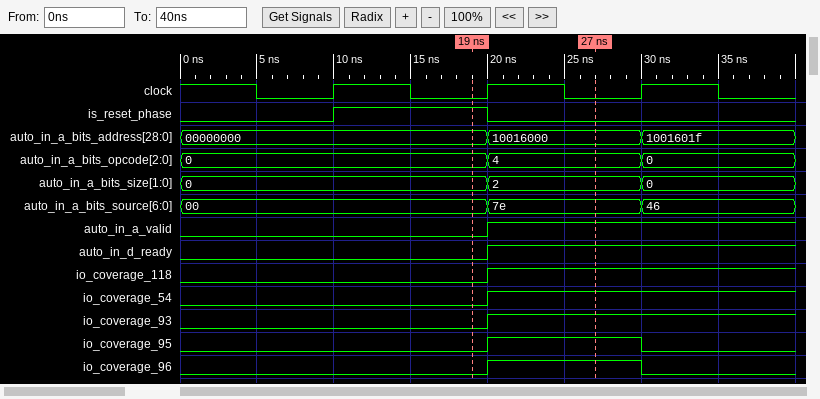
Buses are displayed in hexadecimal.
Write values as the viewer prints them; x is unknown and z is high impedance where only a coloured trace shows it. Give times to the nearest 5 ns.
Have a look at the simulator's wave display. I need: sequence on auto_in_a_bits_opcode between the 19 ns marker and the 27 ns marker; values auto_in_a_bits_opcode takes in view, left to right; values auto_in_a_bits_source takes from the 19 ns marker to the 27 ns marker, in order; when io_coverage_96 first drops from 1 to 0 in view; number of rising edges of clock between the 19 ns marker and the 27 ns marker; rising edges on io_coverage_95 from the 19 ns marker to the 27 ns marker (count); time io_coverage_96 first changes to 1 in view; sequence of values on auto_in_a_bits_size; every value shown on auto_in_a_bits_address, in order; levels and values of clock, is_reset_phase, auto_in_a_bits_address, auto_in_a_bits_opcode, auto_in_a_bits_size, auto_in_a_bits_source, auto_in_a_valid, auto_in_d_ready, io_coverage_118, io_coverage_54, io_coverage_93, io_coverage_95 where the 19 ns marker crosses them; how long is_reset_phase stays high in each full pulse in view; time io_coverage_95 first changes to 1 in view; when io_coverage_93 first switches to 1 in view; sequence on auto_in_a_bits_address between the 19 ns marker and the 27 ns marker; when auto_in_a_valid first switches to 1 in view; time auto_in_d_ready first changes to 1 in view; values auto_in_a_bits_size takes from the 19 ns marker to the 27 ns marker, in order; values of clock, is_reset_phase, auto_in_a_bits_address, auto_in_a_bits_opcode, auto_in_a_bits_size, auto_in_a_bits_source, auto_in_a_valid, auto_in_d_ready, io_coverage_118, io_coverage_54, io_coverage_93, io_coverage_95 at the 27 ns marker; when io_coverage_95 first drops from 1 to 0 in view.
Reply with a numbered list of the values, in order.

1. 0, 4
2. 0, 4, 0
3. 00, 7e
4. 30 ns
5. 1
6. 1
7. 20 ns
8. 0, 2, 0
9. 00000000, 10016000, 1001601f
10. clock=0, is_reset_phase=1, auto_in_a_bits_address=00000000, auto_in_a_bits_opcode=0, auto_in_a_bits_size=0, auto_in_a_bits_source=00, auto_in_a_valid=0, auto_in_d_ready=0, io_coverage_118=0, io_coverage_54=0, io_coverage_93=0, io_coverage_95=0
11. 10 ns
12. 20 ns
13. 20 ns
14. 00000000, 10016000
15. 20 ns
16. 20 ns
17. 0, 2
18. clock=0, is_reset_phase=0, auto_in_a_bits_address=10016000, auto_in_a_bits_opcode=4, auto_in_a_bits_size=2, auto_in_a_bits_source=7e, auto_in_a_valid=1, auto_in_d_ready=1, io_coverage_118=1, io_coverage_54=1, io_coverage_93=1, io_coverage_95=1
19. 30 ns
